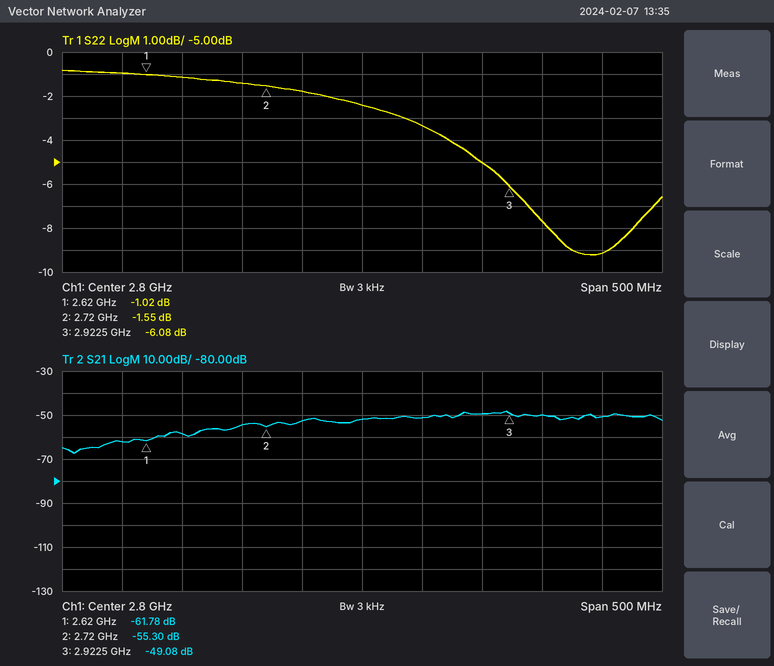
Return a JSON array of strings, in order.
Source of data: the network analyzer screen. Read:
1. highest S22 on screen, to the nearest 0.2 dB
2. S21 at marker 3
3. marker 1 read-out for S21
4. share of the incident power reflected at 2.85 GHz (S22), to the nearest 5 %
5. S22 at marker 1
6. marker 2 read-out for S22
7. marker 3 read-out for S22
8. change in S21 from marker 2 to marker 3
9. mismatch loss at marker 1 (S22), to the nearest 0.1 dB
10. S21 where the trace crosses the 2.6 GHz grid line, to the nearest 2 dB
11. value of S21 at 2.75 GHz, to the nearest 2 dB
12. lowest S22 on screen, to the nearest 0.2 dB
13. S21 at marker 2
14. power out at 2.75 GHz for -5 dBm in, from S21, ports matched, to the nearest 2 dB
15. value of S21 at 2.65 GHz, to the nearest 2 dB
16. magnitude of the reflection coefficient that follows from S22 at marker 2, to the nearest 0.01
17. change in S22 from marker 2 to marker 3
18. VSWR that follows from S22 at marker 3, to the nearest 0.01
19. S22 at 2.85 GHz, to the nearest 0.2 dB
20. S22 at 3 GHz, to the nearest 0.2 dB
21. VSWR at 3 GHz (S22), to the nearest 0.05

["-0.8 dB", "-49.08 dB", "-61.78 dB", "45 %", "-1.02 dB", "-1.55 dB", "-6.08 dB", "6.22 dB", "6.8 dB", "-62 dB", "-52 dB", "-9.2 dB", "-55.30 dB", "-58 dBm", "-58 dB", "0.84", "-4.53 dB", "2.97", "-3.4 dB", "-9.2 dB", "2.05"]
